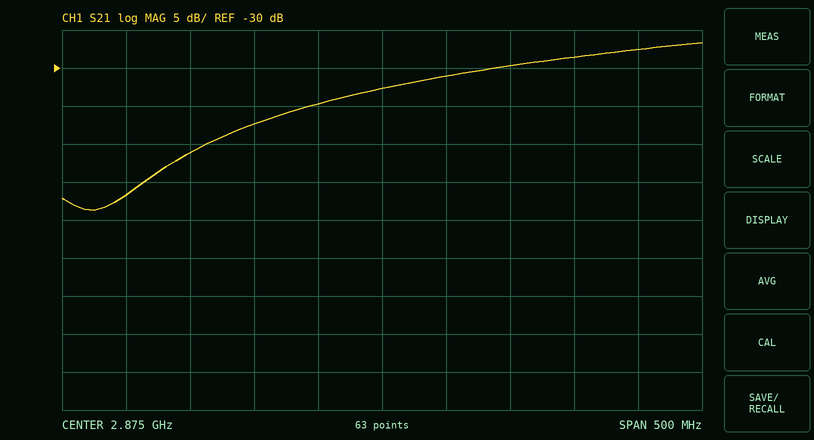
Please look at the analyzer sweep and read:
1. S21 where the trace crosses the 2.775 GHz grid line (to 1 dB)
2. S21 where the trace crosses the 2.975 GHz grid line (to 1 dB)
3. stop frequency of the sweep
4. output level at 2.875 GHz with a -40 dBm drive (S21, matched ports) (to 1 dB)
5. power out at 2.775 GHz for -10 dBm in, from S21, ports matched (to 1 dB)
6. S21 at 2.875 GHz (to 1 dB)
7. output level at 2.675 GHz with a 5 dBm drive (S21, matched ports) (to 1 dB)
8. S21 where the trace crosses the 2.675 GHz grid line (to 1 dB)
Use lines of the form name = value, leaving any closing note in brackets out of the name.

S21 where the trace crosses the 2.775 GHz grid line = -37 dB
S21 where the trace crosses the 2.975 GHz grid line = -30 dB
stop frequency of the sweep = 3.125 GHz
output level at 2.875 GHz with a -40 dBm drive (S21, matched ports) = -73 dBm
power out at 2.775 GHz for -10 dBm in, from S21, ports matched = -47 dBm
S21 at 2.875 GHz = -33 dB
output level at 2.675 GHz with a 5 dBm drive (S21, matched ports) = -42 dBm
S21 where the trace crosses the 2.675 GHz grid line = -47 dB
